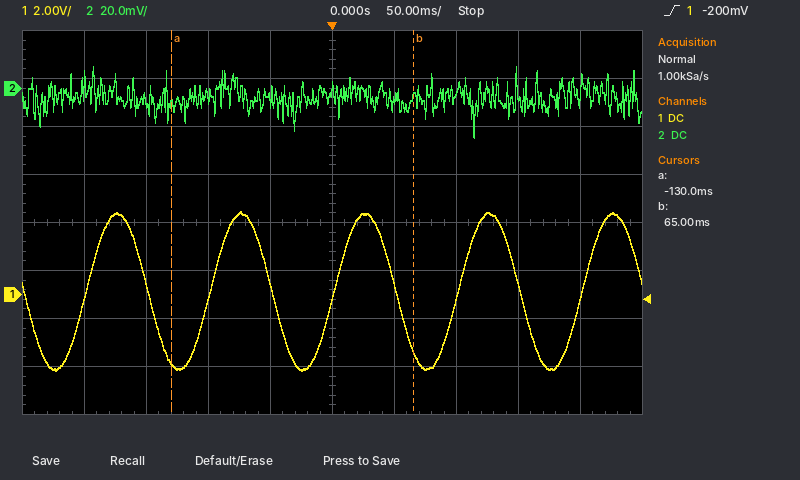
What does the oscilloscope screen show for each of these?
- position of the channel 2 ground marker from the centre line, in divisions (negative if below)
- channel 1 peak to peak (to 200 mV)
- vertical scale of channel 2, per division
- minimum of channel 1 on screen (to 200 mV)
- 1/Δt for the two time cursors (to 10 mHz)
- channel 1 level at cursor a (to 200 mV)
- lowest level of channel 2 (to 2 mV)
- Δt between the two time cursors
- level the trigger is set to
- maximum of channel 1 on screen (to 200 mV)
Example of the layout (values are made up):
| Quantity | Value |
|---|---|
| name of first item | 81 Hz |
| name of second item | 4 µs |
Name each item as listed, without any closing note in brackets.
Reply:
| Quantity | Value |
|---|---|
| position of the channel 2 ground marker from the centre line, in divisions | +2.8 div |
| channel 1 peak to peak | 6.6 V |
| vertical scale of channel 2, per division | 20 mV |
| minimum of channel 1 on screen | -3.2 V |
| 1/Δt for the two time cursors | 5.13 Hz |
| channel 1 level at cursor a | -2.8 V |
| lowest level of channel 2 | -20 mV |
| Δt between the two time cursors | 195 ms |
| level the trigger is set to | -200 mV |
| maximum of channel 1 on screen | 3.4 V |
